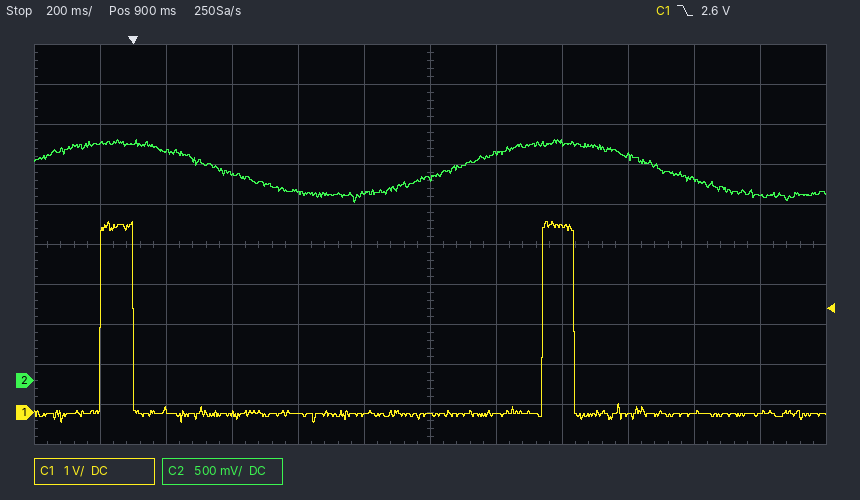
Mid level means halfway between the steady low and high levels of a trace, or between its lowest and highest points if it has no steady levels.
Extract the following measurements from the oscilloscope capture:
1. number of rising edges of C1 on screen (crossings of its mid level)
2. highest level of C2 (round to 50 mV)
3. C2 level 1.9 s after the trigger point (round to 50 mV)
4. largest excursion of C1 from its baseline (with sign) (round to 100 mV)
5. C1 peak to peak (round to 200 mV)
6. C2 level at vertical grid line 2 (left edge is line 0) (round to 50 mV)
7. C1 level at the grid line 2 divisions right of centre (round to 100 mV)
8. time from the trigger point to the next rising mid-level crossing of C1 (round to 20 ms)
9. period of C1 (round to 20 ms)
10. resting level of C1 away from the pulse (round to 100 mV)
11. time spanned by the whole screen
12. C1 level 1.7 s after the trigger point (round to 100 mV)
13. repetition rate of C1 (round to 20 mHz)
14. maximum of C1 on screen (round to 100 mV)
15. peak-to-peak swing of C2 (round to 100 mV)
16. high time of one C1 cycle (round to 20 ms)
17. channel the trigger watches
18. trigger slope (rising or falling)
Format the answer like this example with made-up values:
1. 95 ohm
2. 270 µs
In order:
1. 2
2. 3.00 V
3. 2.30 V
4. +4.8 V
5. 5.0 V
6. 2.85 V
7. 4.7 V
8. 1.24 s
9. 1.34 s
10. 0.0 V
11. 2.4 s
12. 0.0 V
13. 740 mHz
14. 4.8 V
15. 800 mV
16. 100 ms
17. C1
18. falling
